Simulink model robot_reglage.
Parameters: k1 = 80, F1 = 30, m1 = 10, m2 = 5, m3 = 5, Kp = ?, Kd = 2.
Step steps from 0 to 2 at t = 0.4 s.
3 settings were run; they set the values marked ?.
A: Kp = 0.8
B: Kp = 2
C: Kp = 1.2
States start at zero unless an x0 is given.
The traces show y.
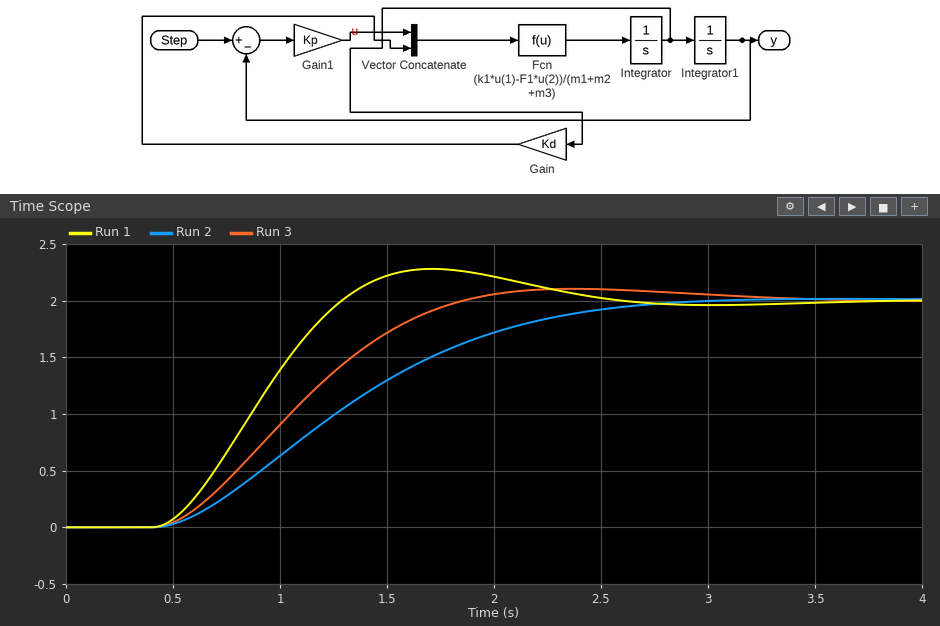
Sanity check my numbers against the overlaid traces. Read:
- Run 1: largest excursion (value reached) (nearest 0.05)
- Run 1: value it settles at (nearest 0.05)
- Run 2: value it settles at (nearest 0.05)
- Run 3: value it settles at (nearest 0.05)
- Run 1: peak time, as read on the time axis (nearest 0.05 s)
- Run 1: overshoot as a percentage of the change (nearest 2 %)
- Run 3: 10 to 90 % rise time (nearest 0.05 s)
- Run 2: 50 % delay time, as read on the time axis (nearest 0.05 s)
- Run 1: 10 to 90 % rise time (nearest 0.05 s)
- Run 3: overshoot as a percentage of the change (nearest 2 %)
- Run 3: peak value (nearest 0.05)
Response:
2.30
2.00
2.00
2.00
1.70 s
14 %
0.95 s
1.25 s
0.60 s
6 %
2.10
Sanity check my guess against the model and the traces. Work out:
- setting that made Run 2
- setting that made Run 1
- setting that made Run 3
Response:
A
B
C
